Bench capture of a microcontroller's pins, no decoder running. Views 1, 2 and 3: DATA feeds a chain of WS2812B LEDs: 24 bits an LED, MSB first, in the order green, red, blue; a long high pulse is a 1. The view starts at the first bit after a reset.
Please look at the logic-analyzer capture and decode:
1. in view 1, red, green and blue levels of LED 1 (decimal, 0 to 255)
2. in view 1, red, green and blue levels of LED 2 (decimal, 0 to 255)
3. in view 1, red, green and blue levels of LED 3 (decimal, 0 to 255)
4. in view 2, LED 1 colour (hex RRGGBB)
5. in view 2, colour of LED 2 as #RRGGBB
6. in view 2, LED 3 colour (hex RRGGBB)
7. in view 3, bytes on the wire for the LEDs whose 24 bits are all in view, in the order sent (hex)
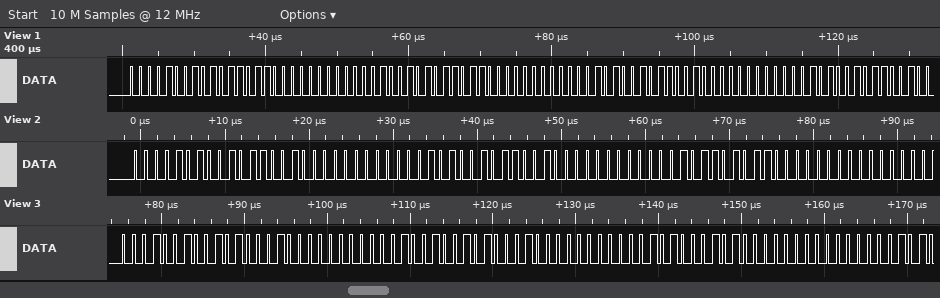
91, 9, 0
91, 9, 0
89, 10, 0
#590A00
#590A00
#580B00
12 51 00 12 51 00 14 50 00
